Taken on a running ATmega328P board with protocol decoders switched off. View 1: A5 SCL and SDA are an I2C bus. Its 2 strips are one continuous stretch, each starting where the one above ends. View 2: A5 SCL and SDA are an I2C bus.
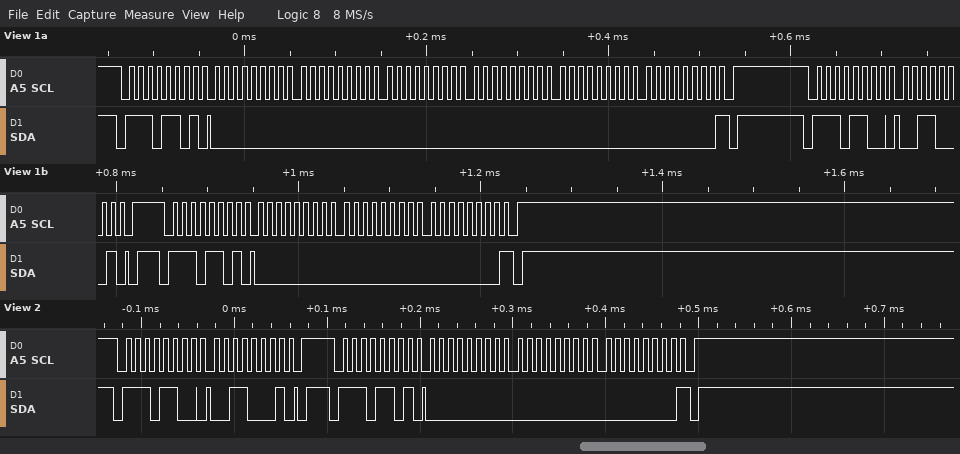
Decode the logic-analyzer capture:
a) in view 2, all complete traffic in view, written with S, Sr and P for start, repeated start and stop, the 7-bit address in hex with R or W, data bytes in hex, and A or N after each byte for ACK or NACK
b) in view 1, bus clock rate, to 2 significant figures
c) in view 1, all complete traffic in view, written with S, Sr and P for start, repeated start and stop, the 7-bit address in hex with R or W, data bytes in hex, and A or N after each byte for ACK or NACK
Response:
S 76W A 31 A P S 76R A 00 A 00 A 00 N P
100 kHz
S 76R A 00 A 00 A 00 A 00 A 00 A 00 N P S 76W A 31 A P S 76R A 00 A 00 A 00 N P
